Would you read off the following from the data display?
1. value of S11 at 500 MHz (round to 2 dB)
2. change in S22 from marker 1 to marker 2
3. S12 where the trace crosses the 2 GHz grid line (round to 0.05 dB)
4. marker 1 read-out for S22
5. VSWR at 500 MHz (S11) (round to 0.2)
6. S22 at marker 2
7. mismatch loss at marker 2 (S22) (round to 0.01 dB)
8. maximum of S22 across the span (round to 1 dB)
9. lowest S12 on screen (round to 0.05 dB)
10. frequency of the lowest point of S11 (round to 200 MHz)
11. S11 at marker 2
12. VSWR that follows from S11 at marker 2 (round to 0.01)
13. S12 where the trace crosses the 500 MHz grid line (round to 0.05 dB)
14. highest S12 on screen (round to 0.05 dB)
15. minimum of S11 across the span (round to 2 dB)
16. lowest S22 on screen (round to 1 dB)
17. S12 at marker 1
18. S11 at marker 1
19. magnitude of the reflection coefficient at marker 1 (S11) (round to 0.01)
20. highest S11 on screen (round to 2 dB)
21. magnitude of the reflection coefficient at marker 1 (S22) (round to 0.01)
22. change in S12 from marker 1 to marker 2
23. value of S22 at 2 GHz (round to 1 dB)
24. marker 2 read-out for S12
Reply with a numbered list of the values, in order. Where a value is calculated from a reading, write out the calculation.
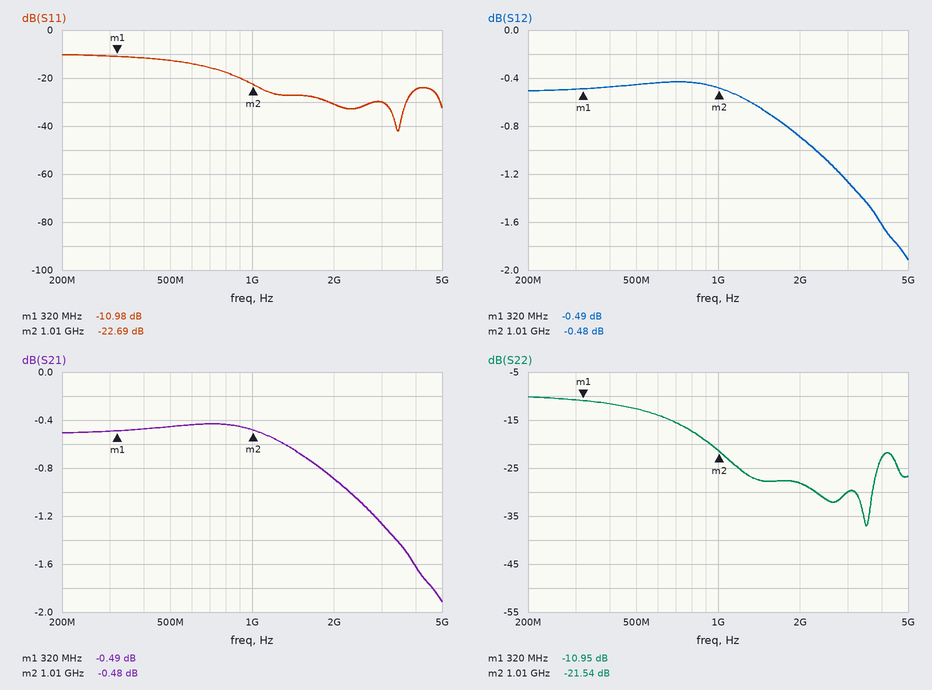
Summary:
1. -12 dB
2. -21.54 − (-10.95) = -10.59 dB
3. -0.90 dB
4. -10.95 dB
5. |Γ| = 10^(-12/20) = 0.2512; VSWR = (1 + 0.2512)/(1 − 0.2512) ≈ 1.67, so 1.6 to the nearest 0.2
6. -21.54 dB
7. −10 log10(1 − 10^(-21.54/10)) ≈ 0.03 dB
8. -10 dB
9. -1.90 dB
10. 3.4 GHz
11. -22.69 dB
12. (1 + 0.0734)/(1 − 0.0734) ≈ 1.16
13. -0.45 dB
14. -0.45 dB
15. -42 dB
16. -37 dB
17. -0.49 dB
18. -10.98 dB
19. 10^(-10.98/20) ≈ 0.28
20. -10 dB
21. 10^(-10.95/20) ≈ 0.28
22. -0.48 − (-0.49) = 0.01 dB
23. -28 dB
24. -0.48 dB
